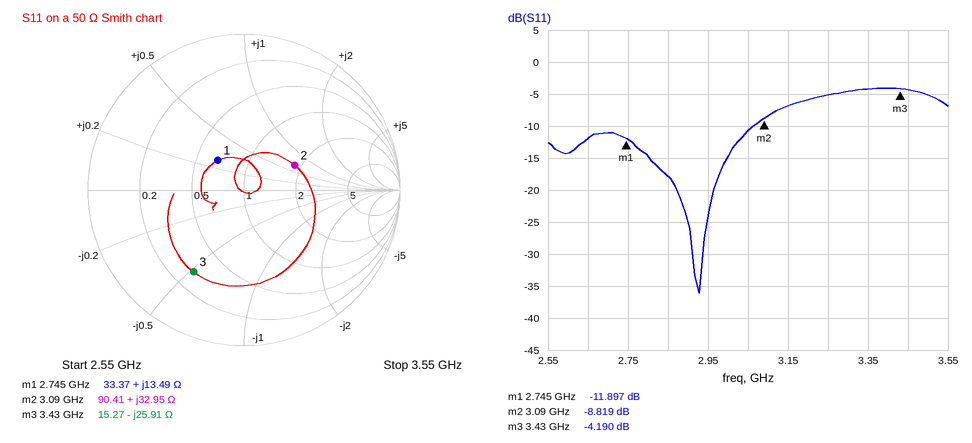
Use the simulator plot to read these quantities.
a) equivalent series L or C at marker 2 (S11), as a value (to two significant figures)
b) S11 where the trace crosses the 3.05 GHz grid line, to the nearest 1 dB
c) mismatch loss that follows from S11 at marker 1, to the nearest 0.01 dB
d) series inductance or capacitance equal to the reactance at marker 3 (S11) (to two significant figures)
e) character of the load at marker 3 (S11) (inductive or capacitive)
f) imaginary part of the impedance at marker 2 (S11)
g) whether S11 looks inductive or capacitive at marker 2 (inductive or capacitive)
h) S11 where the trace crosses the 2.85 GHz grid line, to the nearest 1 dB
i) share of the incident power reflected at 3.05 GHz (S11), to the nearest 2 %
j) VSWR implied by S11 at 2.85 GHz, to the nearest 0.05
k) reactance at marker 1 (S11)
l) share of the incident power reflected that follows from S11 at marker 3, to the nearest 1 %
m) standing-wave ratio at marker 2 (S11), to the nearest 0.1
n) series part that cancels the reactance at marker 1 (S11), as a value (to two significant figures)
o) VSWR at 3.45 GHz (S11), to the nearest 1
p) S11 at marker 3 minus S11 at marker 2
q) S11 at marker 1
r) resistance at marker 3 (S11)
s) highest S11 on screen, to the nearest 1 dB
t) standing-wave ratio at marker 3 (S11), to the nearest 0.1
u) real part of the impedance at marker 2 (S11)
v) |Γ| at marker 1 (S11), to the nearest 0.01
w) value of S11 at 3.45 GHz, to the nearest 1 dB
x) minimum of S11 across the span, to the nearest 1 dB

1.7 nH
-11 dB
0.29 dB
1.8 pF
capacitive
+32.95 Ω
inductive
-18 dB
8 %
1.30
+13.49 Ω
38 %
2.1
4.3 pF
4
4.629 dB
-11.897 dB
15.27 Ω
-4 dB
4.2
90.41 Ω
0.25
-4 dB
-36 dB
